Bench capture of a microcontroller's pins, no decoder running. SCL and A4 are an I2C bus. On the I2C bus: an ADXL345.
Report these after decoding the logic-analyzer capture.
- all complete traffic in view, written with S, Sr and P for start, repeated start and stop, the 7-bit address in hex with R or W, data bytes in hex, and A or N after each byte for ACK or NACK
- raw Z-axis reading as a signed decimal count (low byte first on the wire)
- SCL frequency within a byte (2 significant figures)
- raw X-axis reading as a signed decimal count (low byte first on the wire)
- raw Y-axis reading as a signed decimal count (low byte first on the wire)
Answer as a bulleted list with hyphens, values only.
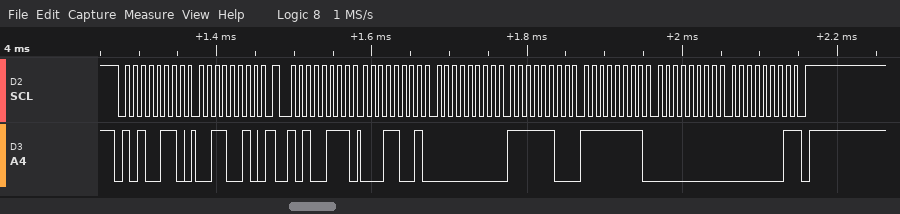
- S 53W A 32 A Sr 53R A 19 A 00 A FC A FF A 00 A 01 N P
- 256
- 100 kHz
- 25
- -4
